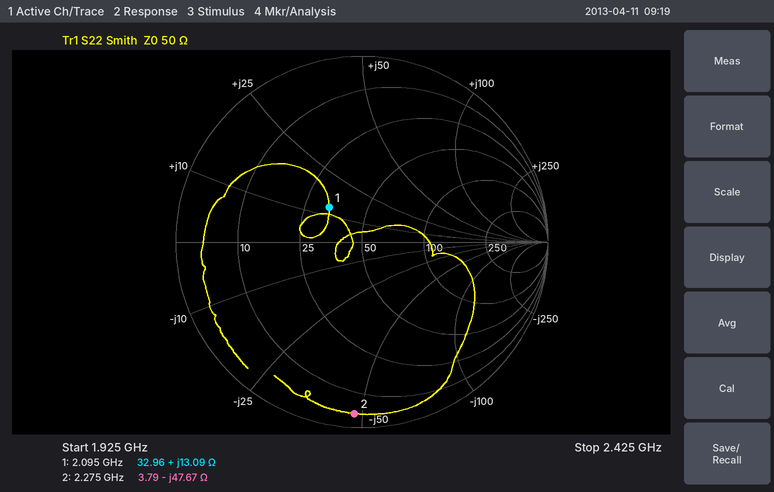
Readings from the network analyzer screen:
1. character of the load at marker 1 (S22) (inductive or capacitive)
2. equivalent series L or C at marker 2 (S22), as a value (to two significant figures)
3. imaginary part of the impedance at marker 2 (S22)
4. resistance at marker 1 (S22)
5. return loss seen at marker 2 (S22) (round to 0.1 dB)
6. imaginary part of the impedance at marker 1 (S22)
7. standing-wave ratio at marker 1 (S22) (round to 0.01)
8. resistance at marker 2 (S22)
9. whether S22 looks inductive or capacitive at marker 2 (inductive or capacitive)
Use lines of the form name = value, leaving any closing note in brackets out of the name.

character of the load at marker 1 (S22) = inductive
equivalent series L or C at marker 2 (S22), as a value = 1.5 pF
imaginary part of the impedance at marker 2 = -47.67 Ω
resistance at marker 1 = 32.96 Ω
return loss seen at marker 2 (S22) = 0.7 dB
imaginary part of the impedance at marker 1 = +13.09 Ω
standing-wave ratio at marker 1 (S22) = 1.69
resistance at marker 2 = 3.79 Ω
whether S22 looks inductive or capacitive at marker 2 = capacitive
